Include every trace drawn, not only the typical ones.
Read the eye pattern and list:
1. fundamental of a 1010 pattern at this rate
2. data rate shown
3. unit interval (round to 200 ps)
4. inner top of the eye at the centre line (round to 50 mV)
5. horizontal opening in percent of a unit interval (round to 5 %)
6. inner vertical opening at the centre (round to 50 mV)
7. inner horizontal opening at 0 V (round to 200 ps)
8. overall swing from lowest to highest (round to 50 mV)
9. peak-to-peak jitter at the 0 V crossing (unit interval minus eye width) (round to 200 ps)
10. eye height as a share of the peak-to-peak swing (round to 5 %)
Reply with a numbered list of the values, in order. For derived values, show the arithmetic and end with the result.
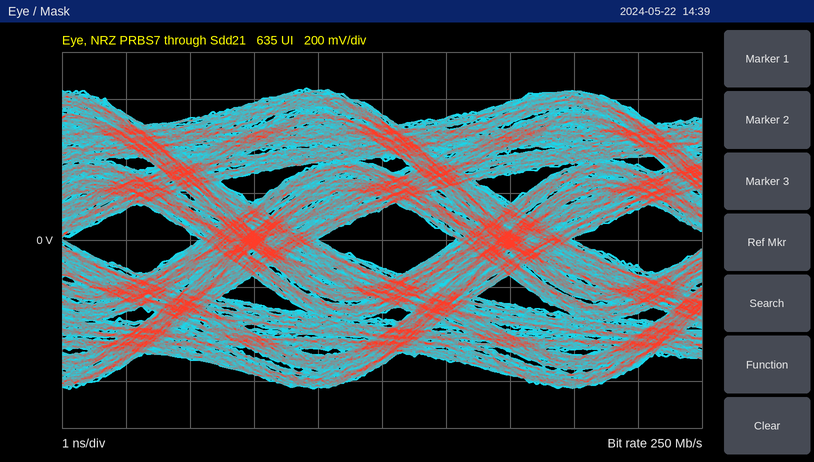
1. 125 MHz
2. 250 Mb/s
3. 4.0 ns
4. 150 mV
5. 2.2 ns / 4.0 ns ≈ 55 %
6. 250 mV
7. 2.2 ns
8. 1.30 V
9. 1.8 ns
10. 250 mV / 1.30 V ≈ 19.2 %, so 20 % to the nearest 5 %
